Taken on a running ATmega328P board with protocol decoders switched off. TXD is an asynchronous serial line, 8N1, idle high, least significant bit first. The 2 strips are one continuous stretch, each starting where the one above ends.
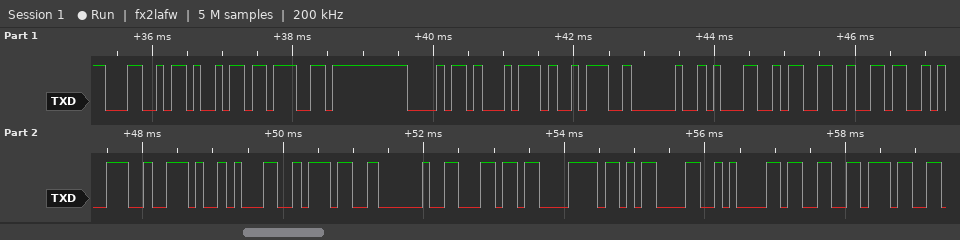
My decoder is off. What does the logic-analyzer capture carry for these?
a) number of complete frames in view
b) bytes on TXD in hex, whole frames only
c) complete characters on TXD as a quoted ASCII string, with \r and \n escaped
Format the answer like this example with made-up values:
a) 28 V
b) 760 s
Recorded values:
a) 21
b) 0x4C 0x69 0x67 0x68 0x74 0x3A 0x20 0x31 0x33 0x36 0x39 0x2E 0x31 0x37 0x20 0x6C 0x78 0x0D 0x0A 0x33 0x37
c) "Light: 1369.17 lx\r\n37"
